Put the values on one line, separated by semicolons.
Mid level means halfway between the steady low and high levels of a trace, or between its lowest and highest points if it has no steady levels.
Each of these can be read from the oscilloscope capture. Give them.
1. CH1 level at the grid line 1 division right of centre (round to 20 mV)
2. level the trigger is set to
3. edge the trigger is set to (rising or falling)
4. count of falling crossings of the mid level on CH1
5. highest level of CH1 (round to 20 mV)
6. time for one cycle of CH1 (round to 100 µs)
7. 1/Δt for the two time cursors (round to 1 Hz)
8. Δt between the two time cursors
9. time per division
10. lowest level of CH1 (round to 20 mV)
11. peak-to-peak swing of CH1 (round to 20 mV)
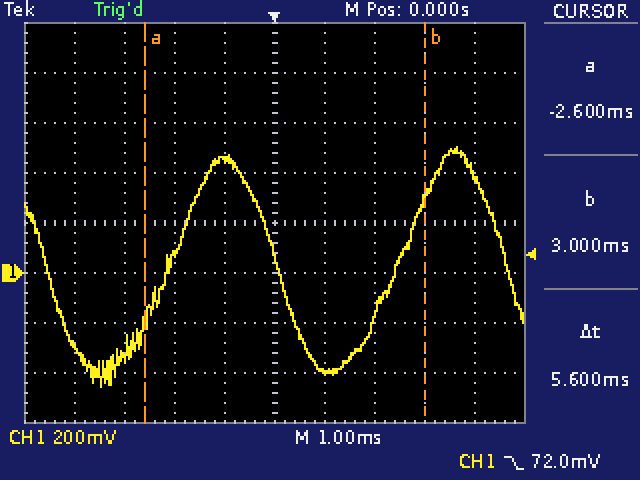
-400 mV; 72.0 mV; falling; 3; 500 mV; 4.6 ms; 179 Hz; 5.6 ms; 1 ms; -460 mV; 960 mV
